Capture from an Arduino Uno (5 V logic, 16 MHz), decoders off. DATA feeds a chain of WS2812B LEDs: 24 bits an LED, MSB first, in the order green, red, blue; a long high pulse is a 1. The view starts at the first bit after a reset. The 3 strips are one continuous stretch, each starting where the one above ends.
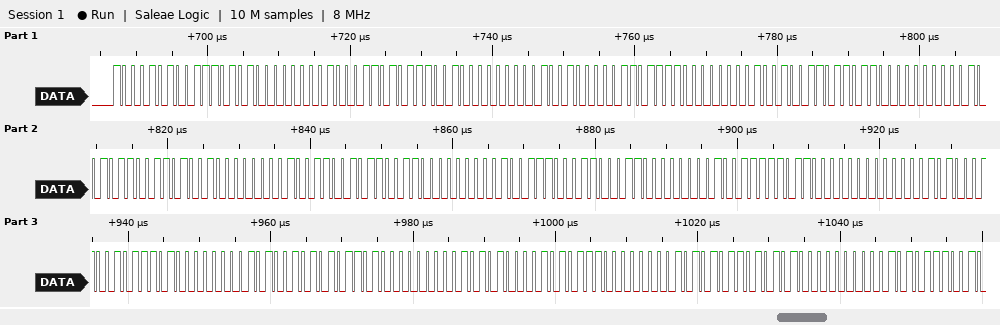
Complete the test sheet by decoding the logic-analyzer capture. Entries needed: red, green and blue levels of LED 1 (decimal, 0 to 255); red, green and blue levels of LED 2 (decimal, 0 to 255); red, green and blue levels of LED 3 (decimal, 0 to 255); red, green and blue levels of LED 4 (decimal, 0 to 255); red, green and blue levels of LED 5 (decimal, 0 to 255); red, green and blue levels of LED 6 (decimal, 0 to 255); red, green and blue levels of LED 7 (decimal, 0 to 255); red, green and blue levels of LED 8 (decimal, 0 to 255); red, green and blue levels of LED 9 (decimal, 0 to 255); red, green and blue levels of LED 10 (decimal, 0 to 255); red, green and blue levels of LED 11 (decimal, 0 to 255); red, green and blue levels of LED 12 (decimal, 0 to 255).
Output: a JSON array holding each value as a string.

["117, 138, 0", "114, 141, 0", "111, 144, 0", "108, 147, 0", "105, 150, 0", "102, 153, 0", "99, 156, 0", "96, 159, 0", "93, 162, 0", "90, 165, 0", "87, 168, 0", "84, 171, 0"]
